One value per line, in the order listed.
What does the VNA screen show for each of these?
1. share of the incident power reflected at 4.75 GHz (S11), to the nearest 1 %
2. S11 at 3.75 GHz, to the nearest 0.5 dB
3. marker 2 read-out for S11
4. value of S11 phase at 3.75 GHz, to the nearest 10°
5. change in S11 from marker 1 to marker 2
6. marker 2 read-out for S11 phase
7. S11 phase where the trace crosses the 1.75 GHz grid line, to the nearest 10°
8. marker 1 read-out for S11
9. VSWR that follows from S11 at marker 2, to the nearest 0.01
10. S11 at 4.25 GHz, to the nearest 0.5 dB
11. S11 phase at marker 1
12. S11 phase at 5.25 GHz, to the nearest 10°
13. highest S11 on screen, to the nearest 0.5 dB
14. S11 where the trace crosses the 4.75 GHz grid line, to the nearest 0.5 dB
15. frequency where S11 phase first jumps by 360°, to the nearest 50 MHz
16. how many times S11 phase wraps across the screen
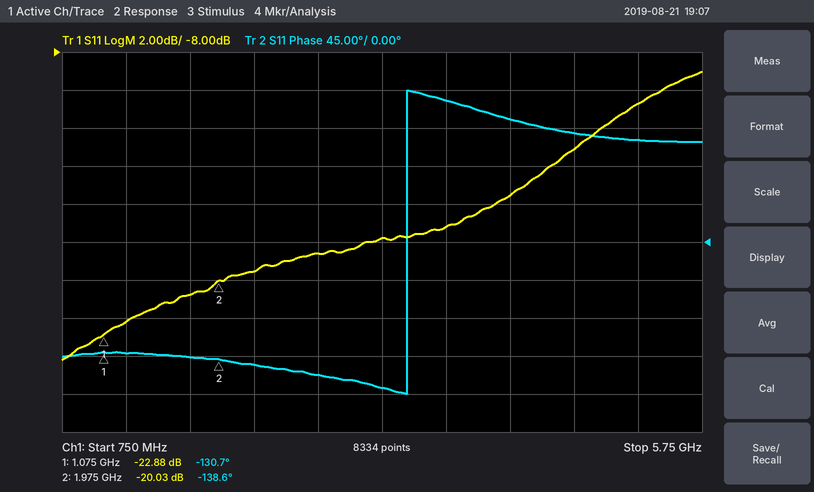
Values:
5 %
-17.0 dB
-20.03 dB
170°
2.85 dB
-138.6°
-140°
-22.88 dB
1.22
-15.5 dB
-130.7°
120°
-9.0 dB
-13.0 dB
3.45 GHz
1
